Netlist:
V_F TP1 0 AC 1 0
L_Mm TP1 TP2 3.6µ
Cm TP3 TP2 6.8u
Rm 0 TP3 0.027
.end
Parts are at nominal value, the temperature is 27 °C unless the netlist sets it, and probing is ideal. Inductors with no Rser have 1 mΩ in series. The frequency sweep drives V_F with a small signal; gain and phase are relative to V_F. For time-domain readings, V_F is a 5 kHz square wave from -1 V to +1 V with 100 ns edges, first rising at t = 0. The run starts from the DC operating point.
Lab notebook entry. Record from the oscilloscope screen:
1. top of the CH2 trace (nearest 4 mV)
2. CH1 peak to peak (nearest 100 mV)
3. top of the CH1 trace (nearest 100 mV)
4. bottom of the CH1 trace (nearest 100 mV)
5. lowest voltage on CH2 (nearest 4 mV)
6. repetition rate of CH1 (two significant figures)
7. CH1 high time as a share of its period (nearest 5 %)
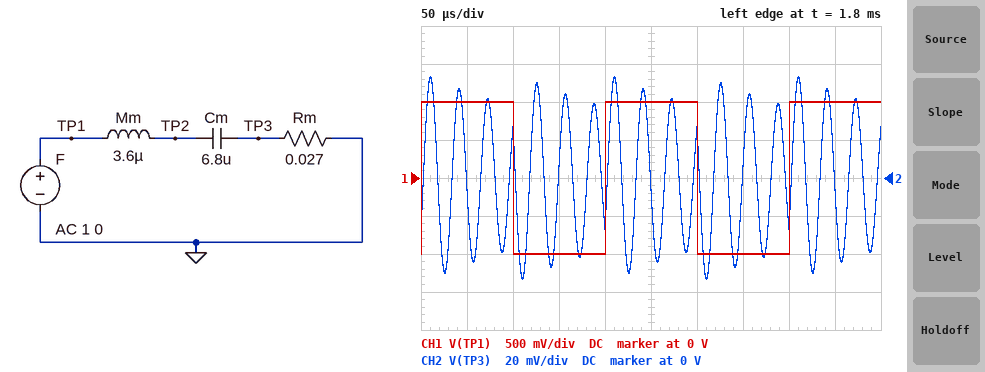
52 mV
2.0 V
1.0 V
-1.0 V
-52 mV
5.0 kHz
50 %
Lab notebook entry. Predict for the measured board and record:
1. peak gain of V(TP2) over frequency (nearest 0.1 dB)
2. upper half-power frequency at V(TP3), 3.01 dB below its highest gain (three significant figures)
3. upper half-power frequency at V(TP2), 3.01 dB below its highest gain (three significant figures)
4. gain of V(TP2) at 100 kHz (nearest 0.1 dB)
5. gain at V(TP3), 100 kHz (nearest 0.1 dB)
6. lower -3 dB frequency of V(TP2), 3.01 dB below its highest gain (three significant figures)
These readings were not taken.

28.3 dB
32.8 kHz
32.8 kHz
-18.7 dB
-37.5 dB
31.5 kHz
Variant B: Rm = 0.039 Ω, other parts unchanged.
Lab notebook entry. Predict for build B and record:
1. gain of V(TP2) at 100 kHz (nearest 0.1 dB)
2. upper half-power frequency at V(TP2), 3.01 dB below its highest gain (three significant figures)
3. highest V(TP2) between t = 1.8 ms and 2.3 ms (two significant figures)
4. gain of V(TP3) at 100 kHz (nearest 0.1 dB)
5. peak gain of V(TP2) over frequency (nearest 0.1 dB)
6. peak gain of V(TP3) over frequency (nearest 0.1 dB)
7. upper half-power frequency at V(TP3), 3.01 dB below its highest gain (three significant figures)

-18.6 dB
33.0 kHz
2.4 V
-34.3 dB
25.2 dB
-0.2 dB
33.1 kHz
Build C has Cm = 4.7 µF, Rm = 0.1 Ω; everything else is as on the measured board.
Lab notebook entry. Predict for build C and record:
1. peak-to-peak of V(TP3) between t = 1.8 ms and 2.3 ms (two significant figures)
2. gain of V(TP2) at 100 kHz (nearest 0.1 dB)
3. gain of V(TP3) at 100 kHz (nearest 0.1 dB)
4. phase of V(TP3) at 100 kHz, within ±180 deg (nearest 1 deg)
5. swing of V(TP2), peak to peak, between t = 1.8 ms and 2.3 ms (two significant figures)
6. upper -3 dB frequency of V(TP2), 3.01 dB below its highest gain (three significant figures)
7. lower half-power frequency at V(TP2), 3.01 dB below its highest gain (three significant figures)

360 mV
-14.7 dB
-25.7 dB
-87 deg
4.9 V
40.7 kHz
36.3 kHz
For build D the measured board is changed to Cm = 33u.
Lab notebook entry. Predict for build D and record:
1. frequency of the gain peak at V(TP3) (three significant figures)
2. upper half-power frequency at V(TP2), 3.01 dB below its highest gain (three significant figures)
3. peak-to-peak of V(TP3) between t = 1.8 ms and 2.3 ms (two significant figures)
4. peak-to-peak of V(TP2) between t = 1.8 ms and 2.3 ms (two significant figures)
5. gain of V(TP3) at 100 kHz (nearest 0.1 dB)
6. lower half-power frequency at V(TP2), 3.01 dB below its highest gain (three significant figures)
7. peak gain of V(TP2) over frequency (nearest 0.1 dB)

14.6 kHz
15.2 kHz
780 mV
11 V
-38.3 dB
13.9 kHz
21.5 dB
